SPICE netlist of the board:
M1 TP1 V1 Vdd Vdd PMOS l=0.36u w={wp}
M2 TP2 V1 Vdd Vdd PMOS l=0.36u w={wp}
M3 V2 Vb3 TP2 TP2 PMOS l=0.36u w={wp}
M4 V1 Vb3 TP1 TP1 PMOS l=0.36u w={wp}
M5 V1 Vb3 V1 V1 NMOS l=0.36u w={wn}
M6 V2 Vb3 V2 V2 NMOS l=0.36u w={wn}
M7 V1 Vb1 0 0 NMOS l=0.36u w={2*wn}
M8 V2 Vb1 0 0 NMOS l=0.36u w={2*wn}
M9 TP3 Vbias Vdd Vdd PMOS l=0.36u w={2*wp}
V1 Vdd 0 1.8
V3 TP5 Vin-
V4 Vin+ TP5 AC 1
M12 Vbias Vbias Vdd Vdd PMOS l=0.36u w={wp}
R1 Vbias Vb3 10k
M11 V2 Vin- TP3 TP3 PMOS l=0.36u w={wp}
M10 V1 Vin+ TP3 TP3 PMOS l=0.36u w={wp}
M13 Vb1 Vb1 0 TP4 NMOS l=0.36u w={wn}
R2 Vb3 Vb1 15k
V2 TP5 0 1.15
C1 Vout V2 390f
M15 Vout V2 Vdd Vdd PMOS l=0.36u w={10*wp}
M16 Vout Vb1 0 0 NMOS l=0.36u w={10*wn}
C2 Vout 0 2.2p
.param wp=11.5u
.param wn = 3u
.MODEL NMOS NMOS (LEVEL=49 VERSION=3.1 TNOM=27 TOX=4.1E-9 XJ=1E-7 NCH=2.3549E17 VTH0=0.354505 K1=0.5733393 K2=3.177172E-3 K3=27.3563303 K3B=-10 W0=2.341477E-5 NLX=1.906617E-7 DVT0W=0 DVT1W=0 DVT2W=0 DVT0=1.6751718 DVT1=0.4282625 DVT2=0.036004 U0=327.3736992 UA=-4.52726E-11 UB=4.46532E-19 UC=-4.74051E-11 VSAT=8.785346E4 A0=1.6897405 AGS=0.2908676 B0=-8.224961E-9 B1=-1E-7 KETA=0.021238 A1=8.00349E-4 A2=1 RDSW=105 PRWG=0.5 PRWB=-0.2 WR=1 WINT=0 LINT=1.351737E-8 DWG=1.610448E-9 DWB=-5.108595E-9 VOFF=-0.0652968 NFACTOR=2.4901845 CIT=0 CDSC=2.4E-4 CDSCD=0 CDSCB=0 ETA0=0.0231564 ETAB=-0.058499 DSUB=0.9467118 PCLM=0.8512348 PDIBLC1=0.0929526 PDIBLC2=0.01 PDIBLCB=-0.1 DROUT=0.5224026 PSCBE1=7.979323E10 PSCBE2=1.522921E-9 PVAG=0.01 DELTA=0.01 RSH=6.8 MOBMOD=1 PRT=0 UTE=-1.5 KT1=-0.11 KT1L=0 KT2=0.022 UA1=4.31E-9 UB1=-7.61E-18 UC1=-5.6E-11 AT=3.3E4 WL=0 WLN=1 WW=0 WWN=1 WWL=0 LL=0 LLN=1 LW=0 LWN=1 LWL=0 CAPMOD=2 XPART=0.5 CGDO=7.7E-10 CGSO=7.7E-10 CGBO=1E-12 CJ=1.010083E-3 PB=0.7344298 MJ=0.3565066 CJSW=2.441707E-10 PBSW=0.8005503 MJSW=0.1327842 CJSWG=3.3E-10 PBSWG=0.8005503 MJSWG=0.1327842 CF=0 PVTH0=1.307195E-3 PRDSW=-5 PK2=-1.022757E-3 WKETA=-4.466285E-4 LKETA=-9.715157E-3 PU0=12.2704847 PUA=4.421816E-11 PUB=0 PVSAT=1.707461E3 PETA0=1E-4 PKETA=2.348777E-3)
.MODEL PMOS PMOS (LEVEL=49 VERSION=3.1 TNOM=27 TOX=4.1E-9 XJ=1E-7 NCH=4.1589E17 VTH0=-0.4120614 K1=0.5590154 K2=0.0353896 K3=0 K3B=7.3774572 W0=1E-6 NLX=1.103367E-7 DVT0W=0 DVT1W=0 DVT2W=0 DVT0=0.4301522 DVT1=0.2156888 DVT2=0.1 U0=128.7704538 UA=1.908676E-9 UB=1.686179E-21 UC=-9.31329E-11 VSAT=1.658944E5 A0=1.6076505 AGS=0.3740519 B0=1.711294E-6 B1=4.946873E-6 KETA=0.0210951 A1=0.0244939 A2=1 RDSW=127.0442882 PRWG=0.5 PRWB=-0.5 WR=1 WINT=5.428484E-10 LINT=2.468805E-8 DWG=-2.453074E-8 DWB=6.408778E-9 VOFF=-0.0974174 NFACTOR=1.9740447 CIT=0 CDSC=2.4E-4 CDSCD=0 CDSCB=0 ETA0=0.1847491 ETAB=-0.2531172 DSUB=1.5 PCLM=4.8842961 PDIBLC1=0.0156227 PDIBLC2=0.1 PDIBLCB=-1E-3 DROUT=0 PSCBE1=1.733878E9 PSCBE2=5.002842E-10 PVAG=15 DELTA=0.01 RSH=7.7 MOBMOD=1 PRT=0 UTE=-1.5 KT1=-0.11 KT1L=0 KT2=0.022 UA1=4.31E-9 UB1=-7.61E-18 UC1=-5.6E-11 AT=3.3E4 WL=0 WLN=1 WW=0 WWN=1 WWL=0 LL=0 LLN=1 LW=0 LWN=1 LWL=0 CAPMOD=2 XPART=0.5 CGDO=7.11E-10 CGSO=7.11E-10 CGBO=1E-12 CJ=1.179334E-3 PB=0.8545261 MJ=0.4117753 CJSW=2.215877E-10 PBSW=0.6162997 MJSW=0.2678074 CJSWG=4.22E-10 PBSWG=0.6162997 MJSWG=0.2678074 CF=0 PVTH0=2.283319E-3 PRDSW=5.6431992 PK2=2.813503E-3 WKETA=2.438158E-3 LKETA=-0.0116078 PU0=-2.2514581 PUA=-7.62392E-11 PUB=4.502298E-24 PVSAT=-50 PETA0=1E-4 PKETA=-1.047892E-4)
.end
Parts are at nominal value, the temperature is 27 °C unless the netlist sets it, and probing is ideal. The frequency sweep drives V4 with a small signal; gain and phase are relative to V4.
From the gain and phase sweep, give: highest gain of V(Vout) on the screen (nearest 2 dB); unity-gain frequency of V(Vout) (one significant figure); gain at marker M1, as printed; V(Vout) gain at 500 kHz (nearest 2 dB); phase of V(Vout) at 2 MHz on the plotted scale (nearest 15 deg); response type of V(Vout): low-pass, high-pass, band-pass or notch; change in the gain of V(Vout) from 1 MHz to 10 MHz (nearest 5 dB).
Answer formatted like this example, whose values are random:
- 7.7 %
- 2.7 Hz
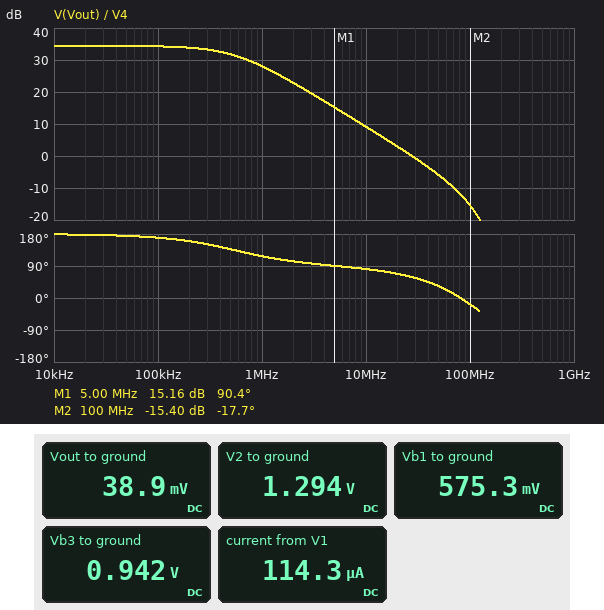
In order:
- 34 dB
- 30 MHz
- 15.16 dB
- 32 dB
- 105 deg
- low-pass
- -20 dB
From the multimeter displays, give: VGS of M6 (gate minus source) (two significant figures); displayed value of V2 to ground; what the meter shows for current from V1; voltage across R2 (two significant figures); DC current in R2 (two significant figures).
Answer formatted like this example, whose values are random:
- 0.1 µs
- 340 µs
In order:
- -350 mV
- 1.294 V
- 114.3 µA
- 370 mV
- 24 µA
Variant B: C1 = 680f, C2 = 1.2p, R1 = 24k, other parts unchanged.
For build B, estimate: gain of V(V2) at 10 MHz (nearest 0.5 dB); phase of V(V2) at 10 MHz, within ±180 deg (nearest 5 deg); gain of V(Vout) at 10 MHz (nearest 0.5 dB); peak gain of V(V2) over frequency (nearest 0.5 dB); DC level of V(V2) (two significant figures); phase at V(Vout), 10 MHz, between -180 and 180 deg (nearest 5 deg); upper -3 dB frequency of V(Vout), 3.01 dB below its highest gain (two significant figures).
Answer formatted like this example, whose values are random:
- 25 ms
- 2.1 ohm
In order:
- 5.0 dB
- -95 deg
- -19.0 dB
- 32.5 dB
- 1.4 V
- 35 deg
- 510 kHz
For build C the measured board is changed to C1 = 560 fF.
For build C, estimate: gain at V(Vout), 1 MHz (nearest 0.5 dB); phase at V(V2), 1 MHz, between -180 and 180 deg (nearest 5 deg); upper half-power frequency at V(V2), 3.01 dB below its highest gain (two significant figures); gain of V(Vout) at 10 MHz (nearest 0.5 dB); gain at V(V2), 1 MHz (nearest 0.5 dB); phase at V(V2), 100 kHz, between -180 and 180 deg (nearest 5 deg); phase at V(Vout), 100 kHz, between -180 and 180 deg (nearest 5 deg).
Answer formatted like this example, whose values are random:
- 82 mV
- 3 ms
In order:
- 26.5 dB
- -65 deg
- 430 kHz
- 7.0 dB
- 26.0 dB
- -15 deg
- 165 deg
